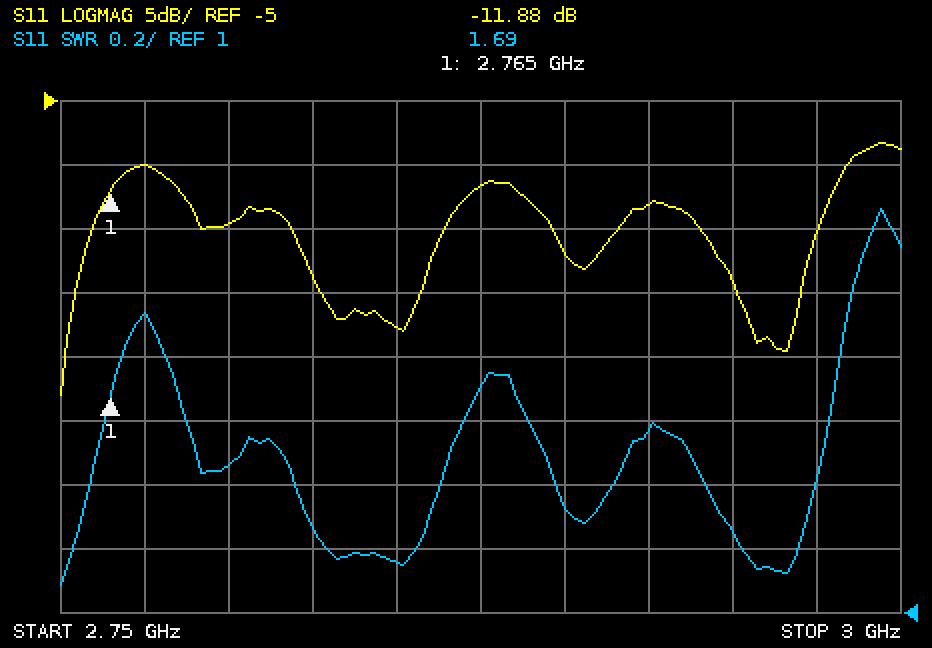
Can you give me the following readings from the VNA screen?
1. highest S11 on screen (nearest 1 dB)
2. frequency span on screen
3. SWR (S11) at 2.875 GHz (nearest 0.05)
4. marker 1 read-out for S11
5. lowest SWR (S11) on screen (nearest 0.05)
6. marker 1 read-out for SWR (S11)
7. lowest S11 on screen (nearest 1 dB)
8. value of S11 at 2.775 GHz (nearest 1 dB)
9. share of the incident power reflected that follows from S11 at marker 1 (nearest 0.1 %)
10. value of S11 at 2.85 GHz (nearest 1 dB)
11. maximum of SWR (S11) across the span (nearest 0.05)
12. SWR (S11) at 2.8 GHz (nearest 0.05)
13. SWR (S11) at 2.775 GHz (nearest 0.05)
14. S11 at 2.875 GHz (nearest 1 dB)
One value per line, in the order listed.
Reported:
-8 dB
250 MHz
1.70
-11.88 dB
1.10
1.69
-28 dB
-10 dB
6.5 %
-23 dB
2.25
1.45
1.95
-12 dB
